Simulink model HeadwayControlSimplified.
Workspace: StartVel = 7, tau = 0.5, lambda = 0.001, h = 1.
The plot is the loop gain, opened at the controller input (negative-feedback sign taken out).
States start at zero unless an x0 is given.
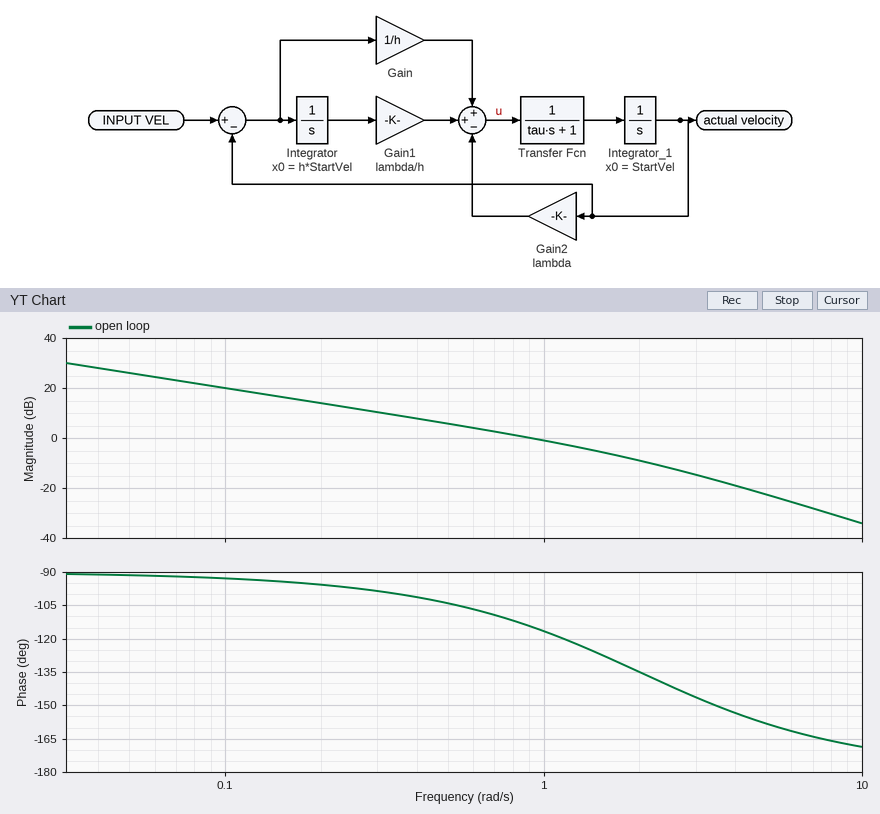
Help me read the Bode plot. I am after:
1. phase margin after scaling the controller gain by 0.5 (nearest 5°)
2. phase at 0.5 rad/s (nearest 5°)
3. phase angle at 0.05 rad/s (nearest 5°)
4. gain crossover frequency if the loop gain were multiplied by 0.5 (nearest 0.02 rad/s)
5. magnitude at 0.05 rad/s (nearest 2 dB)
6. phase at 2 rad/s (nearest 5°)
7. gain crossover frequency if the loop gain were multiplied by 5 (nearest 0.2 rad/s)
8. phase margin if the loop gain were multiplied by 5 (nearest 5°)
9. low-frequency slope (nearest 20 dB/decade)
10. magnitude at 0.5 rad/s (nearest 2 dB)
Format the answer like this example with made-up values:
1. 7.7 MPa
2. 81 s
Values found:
1. 75°
2. -105°
3. -90°
4. 0.48 rad/s
5. 26 dB
6. -135°
7. 2.8 rad/s
8. 35°
9. -20 dB/decade
10. 6 dB
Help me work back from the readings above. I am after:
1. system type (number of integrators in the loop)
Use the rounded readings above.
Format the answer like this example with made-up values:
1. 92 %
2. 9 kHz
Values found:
1. 1
